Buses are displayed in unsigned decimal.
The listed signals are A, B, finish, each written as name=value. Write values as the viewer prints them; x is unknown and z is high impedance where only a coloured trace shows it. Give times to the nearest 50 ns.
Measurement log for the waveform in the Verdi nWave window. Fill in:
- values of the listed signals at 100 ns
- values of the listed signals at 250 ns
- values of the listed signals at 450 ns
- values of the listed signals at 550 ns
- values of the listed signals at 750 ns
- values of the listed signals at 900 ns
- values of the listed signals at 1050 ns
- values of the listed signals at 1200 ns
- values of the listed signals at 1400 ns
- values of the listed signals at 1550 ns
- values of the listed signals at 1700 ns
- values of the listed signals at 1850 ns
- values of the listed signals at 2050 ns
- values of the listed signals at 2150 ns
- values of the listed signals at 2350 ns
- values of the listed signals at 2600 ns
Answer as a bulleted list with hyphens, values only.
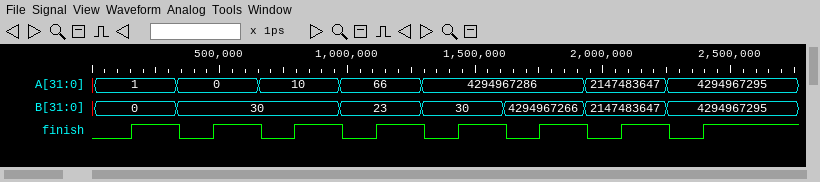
- A=1, B=0, finish=0
- A=1, B=0, finish=1
- A=0, B=30, finish=0
- A=0, B=30, finish=1
- A=10, B=30, finish=0
- A=10, B=30, finish=1
- A=66, B=23, finish=0
- A=66, B=23, finish=1
- A=4294967286, B=30, finish=0
- A=4294967286, B=30, finish=1
- A=4294967286, B=4294967266, finish=0
- A=4294967286, B=4294967266, finish=1
- A=2147483647, B=2147483647, finish=0
- A=2147483647, B=2147483647, finish=1
- A=4294967295, B=4294967295, finish=0
- A=4294967295, B=4294967295, finish=1
